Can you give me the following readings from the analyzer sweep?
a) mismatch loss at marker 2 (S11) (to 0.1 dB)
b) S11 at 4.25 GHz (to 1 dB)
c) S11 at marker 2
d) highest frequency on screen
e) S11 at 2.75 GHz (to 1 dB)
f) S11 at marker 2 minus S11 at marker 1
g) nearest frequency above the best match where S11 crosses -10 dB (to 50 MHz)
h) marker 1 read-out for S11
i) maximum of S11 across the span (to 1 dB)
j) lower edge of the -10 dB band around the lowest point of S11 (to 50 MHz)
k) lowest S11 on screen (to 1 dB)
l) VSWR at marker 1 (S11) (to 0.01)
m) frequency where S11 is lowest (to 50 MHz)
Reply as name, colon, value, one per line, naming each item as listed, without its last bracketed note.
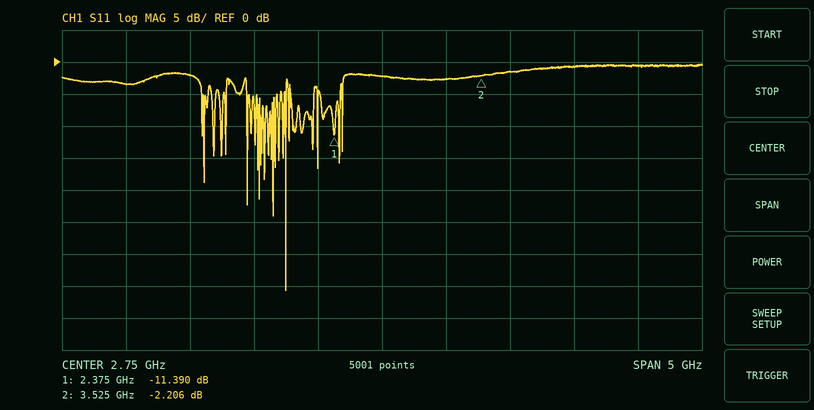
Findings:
mismatch loss at marker 2 (S11): 4.0 dB
S11 at 4.25 GHz: -1 dB
S11 at marker 2: -2.206 dB
highest frequency on screen: 5.25 GHz
S11 at 2.75 GHz: -2 dB
S11 at marker 2 minus S11 at marker 1: 9.184 dB
nearest frequency above the best match where S11 crosses -10 dB: 2.00 GHz
marker 1 read-out for S11: -11.390 dB
maximum of S11 across the span: 0 dB
lower edge of the -10 dB band around the lowest point of S11: 2.00 GHz
lowest S11 on screen: -36 dB
VSWR at marker 1 (S11): 1.74
frequency where S11 is lowest: 2.00 GHz
